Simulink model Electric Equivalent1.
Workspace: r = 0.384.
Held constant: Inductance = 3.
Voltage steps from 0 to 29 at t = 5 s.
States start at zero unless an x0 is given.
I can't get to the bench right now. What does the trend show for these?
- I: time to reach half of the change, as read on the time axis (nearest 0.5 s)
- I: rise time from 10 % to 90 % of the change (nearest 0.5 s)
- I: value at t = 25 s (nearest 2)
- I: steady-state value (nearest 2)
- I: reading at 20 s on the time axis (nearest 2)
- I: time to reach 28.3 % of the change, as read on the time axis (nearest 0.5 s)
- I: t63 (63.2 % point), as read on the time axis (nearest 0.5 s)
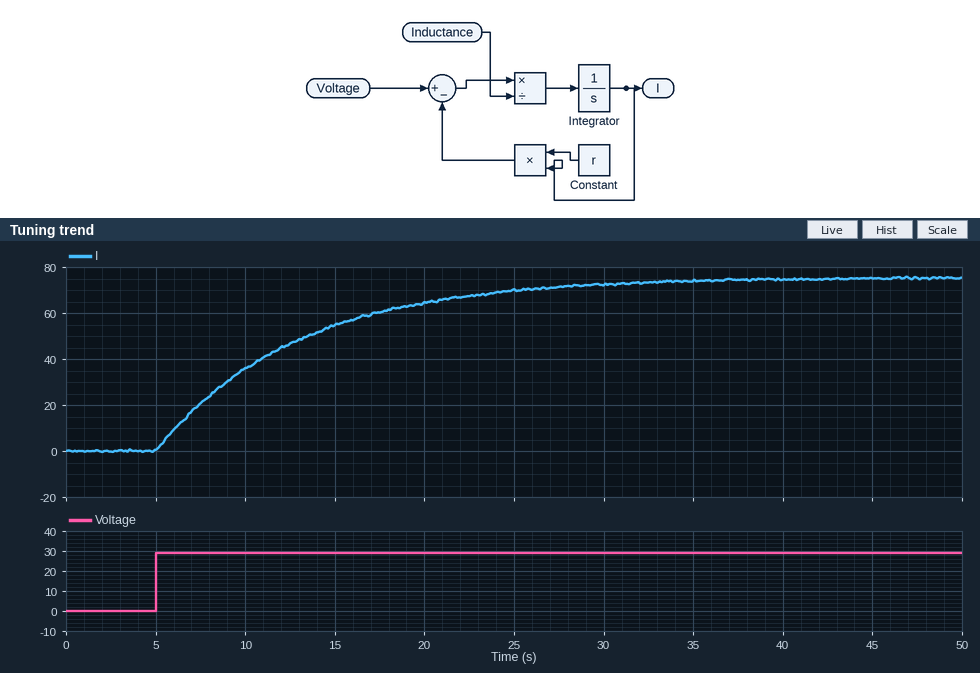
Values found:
10.5 s
17.0 s
70
76
64
7.5 s
13.0 s
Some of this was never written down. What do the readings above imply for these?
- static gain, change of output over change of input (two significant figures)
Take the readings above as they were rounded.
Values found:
2.6
